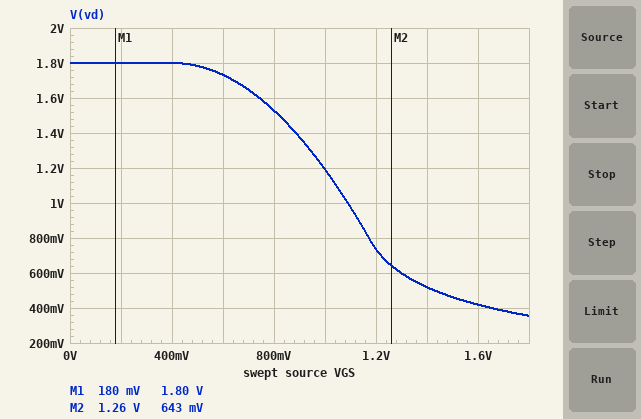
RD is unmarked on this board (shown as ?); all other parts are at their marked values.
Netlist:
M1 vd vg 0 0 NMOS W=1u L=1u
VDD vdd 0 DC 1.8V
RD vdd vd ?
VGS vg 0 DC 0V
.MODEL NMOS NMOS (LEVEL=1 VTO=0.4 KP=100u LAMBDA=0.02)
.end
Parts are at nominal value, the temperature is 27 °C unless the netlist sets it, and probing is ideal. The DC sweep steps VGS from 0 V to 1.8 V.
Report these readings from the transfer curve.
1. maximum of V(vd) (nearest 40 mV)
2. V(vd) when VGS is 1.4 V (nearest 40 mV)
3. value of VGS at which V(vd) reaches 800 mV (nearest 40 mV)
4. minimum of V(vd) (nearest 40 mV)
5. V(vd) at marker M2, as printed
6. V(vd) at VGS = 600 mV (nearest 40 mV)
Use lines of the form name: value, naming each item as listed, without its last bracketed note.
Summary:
maximum of V(vd): 1.80 V
V(vd) when VGS is 1.4 V: 520 mV
value of VGS at which V(vd) reaches 800 mV: 1.16 V
minimum of V(vd): 360 mV
V(vd) at marker M2, as printed: 643 mV
V(vd) at VGS = 600 mV: 1.72 V
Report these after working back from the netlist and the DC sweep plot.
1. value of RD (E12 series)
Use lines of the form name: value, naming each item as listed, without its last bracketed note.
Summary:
value of RD: 33 kΩ
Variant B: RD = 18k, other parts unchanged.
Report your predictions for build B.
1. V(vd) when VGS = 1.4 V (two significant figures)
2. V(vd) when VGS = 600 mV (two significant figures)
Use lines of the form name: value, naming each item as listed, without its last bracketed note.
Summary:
V(vd) when VGS = 1.4 V: 890 mV
V(vd) when VGS = 600 mV: 1.8 V
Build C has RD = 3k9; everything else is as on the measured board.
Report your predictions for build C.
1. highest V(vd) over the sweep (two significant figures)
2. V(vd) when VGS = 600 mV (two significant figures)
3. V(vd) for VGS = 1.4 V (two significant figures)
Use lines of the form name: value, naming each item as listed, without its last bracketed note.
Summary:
highest V(vd) over the sweep: 1.8 V
V(vd) when VGS = 600 mV: 1.8 V
V(vd) for VGS = 1.4 V: 1.6 V
